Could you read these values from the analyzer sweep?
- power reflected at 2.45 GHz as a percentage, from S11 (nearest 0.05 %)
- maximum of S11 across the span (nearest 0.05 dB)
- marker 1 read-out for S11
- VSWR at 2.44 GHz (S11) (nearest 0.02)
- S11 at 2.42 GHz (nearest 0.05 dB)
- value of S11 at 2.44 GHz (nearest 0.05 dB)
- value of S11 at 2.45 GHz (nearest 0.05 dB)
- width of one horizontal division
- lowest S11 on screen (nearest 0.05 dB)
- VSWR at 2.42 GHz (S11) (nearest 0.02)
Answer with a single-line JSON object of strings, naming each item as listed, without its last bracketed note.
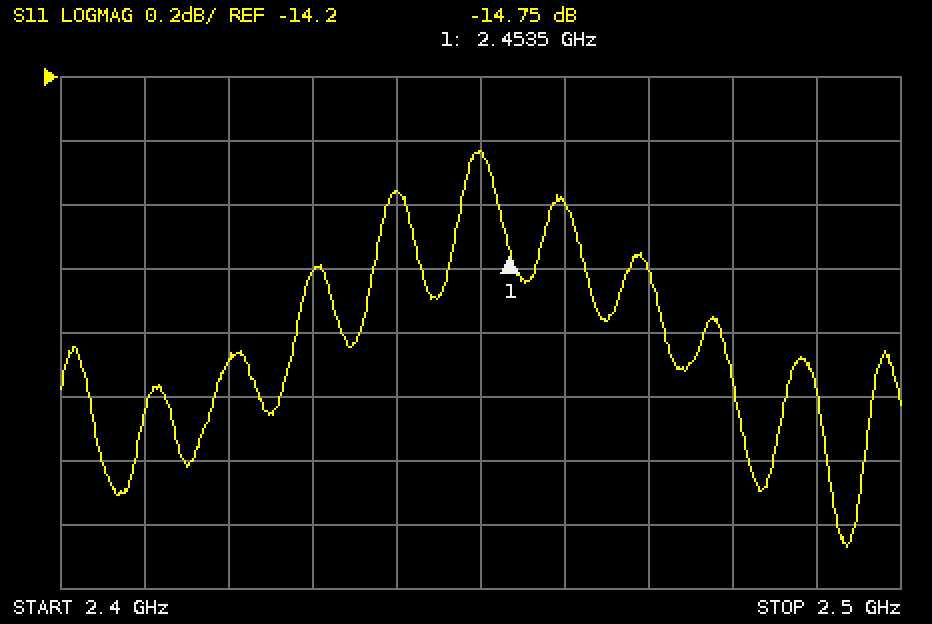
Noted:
{"power reflected at 2.45 GHz as a percentage, from S11": "3.60 %", "maximum of S11 across the span": "-14.45 dB", "marker 1 read-out for S11": "-14.75 dB", "VSWR at 2.44 GHz (S11)": "1.46", "S11 at 2.42 GHz": "-15.10 dB", "value of S11 at 2.44 GHz": "-14.55 dB", "value of S11 at 2.45 GHz": "-14.45 dB", "width of one horizontal division": "10 MHz", "lowest S11 on screen": "-15.65 dB", "VSWR at 2.42 GHz (S11)": "1.42"}
